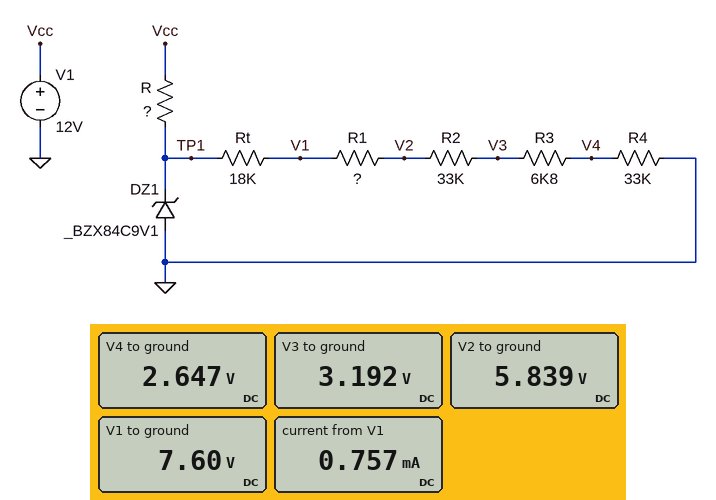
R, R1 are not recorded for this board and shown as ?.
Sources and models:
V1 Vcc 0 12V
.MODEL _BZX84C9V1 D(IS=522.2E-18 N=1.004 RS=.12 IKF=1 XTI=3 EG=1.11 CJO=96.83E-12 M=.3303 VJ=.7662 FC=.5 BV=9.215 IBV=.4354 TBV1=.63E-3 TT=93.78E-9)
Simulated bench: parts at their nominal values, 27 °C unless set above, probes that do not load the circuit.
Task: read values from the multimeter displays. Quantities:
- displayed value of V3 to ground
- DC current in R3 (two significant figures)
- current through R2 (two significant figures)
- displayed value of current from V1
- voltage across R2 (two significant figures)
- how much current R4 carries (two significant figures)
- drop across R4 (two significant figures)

3.192 V
80 µA
80 µA
0.757 mA
2.6 V
80 µA
2.6 V
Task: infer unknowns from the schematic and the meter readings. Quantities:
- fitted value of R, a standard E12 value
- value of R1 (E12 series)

3.9 kΩ
22 kΩ
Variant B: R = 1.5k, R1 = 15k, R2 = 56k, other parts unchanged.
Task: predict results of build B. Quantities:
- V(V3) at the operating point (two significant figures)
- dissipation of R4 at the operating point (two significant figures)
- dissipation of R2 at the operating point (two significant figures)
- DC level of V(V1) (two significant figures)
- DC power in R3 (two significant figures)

2.8 V
160 µW
280 µW
7.8 V
34 µW
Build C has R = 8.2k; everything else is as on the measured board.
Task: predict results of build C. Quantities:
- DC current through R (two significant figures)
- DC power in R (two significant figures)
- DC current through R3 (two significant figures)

360 µA
1.1 mW
80 µA
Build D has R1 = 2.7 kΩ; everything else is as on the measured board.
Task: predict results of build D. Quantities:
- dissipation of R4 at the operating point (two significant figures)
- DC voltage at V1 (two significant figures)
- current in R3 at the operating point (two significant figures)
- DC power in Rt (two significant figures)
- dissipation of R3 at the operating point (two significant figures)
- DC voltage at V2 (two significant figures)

310 µW
7.3 V
97 µA
170 µW
64 µW
7.0 V
